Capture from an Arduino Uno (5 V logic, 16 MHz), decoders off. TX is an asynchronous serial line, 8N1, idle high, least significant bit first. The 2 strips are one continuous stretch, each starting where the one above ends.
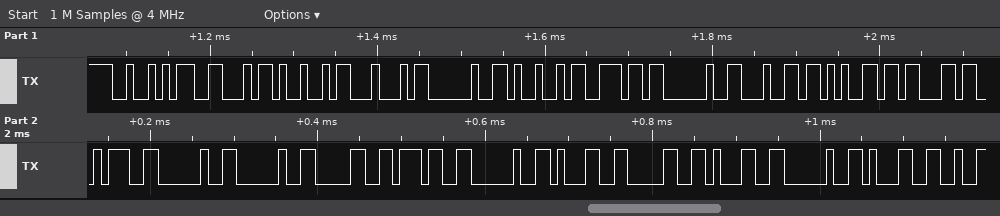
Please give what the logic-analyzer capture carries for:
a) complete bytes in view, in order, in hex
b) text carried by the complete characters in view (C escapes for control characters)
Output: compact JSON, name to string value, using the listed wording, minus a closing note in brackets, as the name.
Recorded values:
{"complete bytes in view, in order, in hex": "52 46 49 44 20 49 6E 20 64 65 63 3A 20 20 30 37 20 31 30 31 20 31", "text carried by the complete characters in view": "\"RFID In dec:  07 101 1\""}
